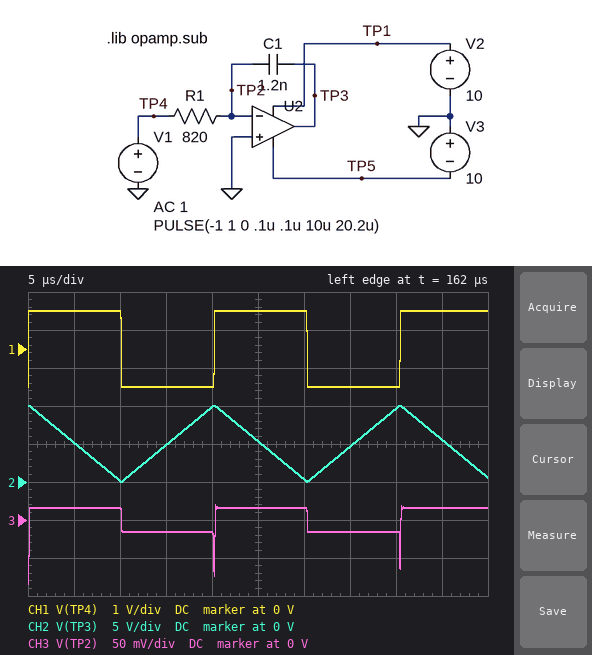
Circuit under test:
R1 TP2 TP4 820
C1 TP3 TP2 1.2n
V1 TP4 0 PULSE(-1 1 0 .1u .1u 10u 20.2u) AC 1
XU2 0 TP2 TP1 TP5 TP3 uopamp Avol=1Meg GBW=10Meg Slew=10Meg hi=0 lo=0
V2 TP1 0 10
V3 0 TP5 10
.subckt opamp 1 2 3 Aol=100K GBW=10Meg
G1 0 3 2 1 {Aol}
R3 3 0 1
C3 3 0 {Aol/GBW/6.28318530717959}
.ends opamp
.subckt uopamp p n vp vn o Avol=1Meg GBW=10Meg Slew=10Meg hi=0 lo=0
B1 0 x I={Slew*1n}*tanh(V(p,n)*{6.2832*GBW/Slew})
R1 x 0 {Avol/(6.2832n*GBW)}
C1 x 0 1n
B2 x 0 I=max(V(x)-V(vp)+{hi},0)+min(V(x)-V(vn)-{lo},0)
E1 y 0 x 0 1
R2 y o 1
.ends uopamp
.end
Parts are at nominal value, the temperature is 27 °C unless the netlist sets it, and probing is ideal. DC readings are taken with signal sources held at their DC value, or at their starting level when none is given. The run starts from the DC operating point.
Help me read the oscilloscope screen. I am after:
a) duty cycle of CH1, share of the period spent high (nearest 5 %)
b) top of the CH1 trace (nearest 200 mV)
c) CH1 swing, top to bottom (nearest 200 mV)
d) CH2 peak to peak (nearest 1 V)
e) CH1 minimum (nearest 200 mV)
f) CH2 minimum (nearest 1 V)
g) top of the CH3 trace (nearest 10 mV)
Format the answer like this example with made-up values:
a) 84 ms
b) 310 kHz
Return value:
a) 50 %
b) 1.0 V
c) 2.0 V
d) 10 V
e) -1.0 V
f) 0 V
g) 20 mV
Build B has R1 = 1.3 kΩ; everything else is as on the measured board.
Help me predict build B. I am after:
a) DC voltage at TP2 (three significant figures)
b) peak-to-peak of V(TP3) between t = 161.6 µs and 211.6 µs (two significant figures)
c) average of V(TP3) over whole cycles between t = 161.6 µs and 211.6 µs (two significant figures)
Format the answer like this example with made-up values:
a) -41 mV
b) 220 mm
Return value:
a) -1.00 V
b) 6.3 V
c) 6.9 V
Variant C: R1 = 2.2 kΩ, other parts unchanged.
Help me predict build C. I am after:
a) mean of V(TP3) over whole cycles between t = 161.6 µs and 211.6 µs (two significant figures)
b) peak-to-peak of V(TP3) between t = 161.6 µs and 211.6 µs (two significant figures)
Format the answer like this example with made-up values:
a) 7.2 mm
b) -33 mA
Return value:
a) 8.2 V
b) 3.7 V
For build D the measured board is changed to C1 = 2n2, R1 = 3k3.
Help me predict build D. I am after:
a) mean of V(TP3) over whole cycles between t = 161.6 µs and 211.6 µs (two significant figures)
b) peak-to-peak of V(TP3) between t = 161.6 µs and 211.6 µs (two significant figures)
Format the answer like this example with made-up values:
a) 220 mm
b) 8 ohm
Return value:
a) 9.4 V
b) 1.3 V
